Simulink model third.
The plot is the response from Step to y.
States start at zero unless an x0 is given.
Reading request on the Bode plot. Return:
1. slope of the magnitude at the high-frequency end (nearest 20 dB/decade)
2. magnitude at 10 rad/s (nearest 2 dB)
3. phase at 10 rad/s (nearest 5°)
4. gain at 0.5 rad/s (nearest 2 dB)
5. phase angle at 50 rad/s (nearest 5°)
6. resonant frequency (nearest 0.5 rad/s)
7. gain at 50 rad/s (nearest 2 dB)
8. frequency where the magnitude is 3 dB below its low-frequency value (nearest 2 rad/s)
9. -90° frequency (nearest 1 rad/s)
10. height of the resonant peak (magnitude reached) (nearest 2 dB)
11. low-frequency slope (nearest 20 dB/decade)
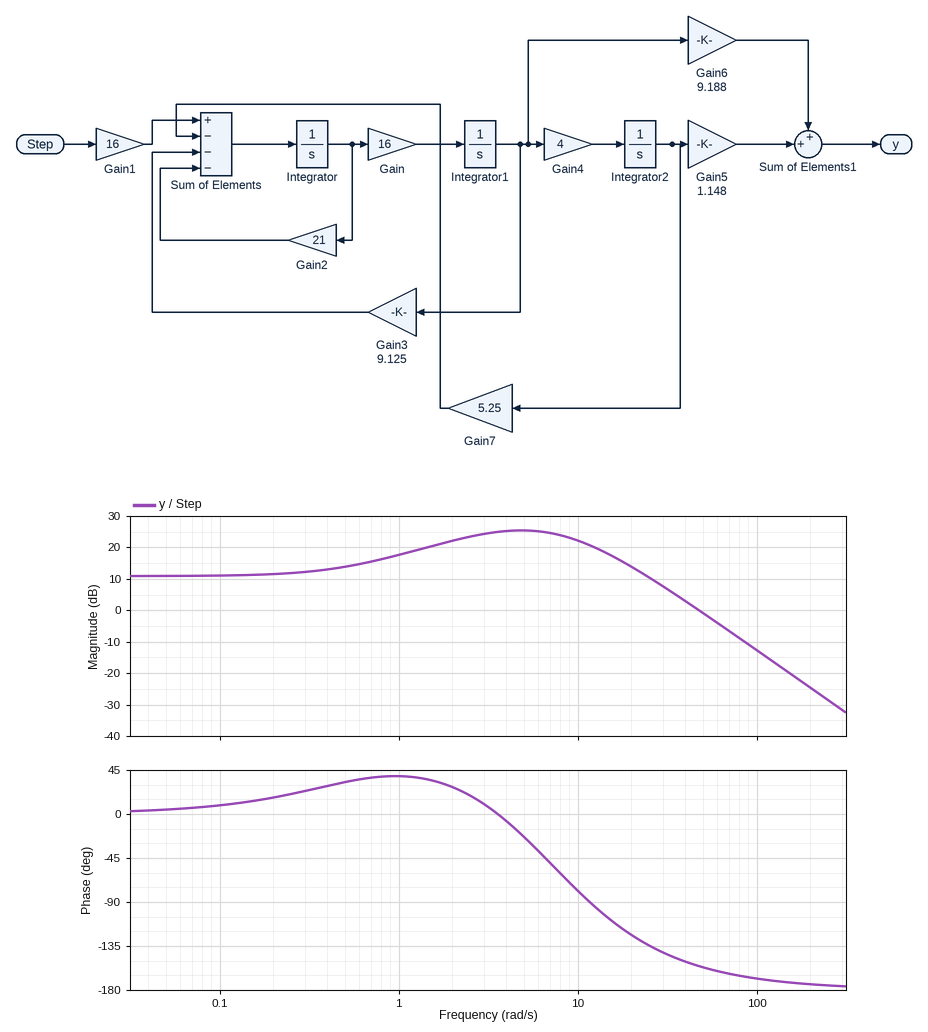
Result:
-40 dB/decade
22 dB
-80°
14 dB
-155°
5.0 rad/s
0 dB
30 rad/s
12 rad/s
26 dB
0 dB/decade
